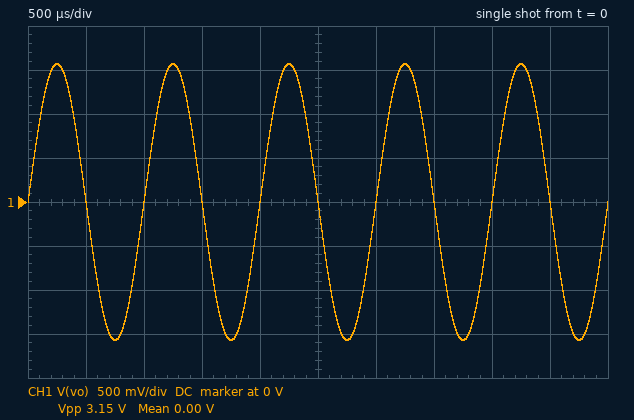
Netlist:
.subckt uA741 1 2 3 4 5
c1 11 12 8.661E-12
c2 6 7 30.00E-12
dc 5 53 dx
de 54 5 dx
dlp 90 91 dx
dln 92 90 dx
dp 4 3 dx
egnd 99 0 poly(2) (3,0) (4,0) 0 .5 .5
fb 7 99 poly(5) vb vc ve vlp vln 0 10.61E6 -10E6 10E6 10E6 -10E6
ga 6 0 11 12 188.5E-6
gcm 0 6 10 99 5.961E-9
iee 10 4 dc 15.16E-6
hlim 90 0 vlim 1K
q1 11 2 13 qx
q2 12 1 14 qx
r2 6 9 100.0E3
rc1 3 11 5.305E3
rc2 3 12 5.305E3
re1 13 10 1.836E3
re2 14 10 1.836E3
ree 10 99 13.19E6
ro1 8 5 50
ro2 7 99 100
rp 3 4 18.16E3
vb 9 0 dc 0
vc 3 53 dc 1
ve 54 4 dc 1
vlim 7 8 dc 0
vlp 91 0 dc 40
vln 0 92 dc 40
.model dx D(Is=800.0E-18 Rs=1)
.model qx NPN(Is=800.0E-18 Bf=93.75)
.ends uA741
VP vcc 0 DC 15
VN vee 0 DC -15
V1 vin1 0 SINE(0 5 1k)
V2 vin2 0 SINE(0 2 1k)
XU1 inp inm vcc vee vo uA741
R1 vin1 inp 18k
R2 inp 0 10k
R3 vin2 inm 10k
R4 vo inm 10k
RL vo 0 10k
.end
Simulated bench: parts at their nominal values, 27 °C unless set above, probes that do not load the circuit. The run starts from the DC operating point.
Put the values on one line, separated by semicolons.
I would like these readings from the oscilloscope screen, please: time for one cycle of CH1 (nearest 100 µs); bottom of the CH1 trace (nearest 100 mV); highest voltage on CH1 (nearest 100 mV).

1.0 ms; -1.6 V; 1.6 V
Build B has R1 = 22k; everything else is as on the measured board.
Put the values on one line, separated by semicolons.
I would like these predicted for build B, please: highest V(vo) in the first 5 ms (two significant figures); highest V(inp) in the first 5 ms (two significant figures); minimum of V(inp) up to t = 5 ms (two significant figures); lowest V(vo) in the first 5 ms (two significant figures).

1.1 V; 1.6 V; -1.6 V; -1.1 V
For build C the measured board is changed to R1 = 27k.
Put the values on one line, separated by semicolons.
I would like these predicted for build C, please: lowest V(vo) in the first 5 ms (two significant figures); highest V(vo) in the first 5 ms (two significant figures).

-700 mV; 700 mV
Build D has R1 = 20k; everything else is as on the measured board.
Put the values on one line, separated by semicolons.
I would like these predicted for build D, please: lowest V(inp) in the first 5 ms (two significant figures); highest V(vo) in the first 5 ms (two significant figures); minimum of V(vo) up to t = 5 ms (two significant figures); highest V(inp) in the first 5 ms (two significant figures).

-1.7 V; 1.3 V; -1.3 V; 1.7 V
